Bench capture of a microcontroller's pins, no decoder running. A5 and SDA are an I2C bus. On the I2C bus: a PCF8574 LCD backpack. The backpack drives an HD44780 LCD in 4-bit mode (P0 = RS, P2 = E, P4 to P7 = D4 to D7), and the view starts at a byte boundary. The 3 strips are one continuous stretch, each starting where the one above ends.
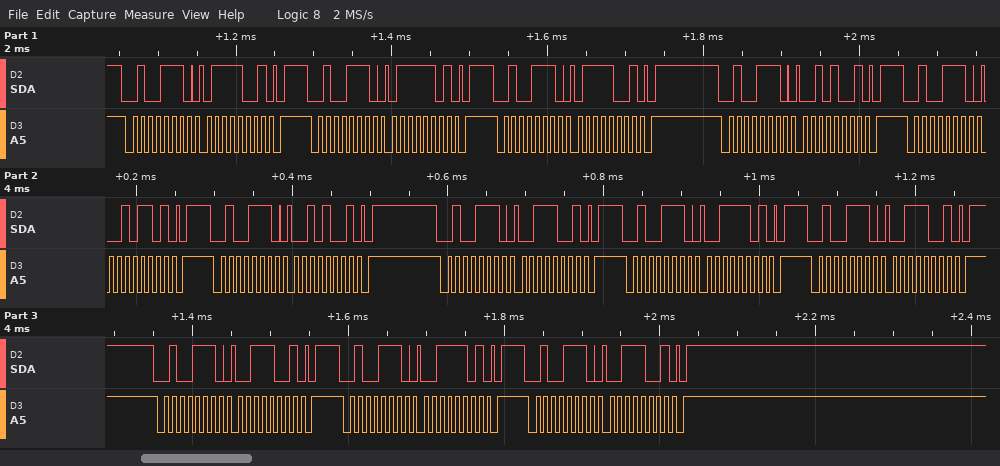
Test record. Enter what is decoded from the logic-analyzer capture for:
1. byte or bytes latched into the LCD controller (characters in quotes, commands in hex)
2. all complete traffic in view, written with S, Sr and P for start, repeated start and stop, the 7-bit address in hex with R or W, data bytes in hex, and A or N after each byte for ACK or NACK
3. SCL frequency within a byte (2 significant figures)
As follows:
'r' '3'
S 27W A 79 A P S 27W A 7D A P S 27W A 79 A P S 27W A 29 A P S 27W A 2D A P S 27W A 29 A P S 27W A 39 A P S 27W A 3D A P S 27W A 39 A P S 27W A 39 A P S 27W A 3D A P S 27W A 39 A P
100 kHz
